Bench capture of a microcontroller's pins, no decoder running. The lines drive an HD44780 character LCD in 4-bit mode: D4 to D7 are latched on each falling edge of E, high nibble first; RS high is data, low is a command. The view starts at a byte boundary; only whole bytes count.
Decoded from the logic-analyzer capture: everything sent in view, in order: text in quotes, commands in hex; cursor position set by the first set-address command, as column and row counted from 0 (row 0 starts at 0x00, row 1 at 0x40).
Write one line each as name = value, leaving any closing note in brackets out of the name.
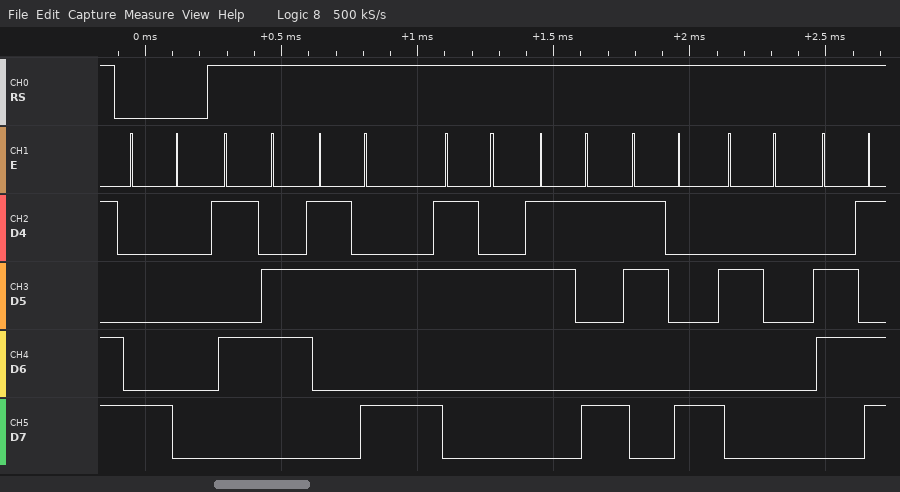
everything sent in view, in order: text in quotes, commands in hex = 0x80 "V:298 m"
cursor position set by the first set-address command, as column and row counted from 0 = column 0, row 0
